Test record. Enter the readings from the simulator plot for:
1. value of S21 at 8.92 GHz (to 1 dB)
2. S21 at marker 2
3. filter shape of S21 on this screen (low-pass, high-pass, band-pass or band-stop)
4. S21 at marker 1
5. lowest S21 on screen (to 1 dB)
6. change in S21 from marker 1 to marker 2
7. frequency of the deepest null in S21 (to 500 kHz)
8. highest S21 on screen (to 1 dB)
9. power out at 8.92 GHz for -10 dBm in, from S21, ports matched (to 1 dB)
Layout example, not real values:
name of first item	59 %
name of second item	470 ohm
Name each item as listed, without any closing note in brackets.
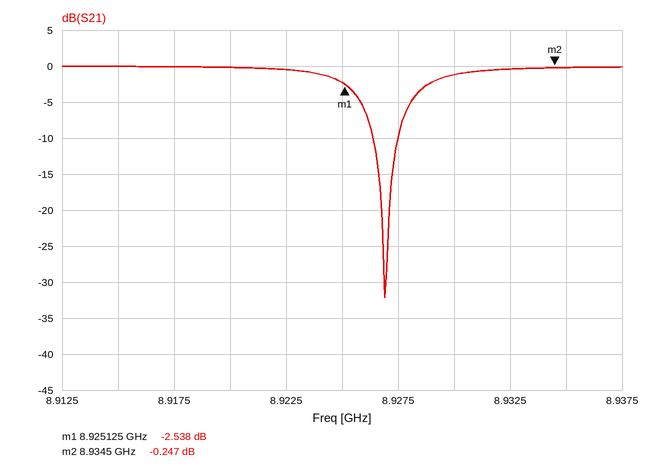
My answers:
value of S21 at 8.92 GHz	0 dB
S21 at marker 2	-0.247 dB
filter shape of S21 on this screen	band-stop
S21 at marker 1	-2.538 dB
lowest S21 on screen	-32 dB
change in S21 from marker 1 to marker 2	2.291 dB
frequency of the deepest null in S21	8.9270 GHz
highest S21 on screen	0 dB
power out at 8.92 GHz for -10 dBm in, from S21, ports matched	-10 dBm
